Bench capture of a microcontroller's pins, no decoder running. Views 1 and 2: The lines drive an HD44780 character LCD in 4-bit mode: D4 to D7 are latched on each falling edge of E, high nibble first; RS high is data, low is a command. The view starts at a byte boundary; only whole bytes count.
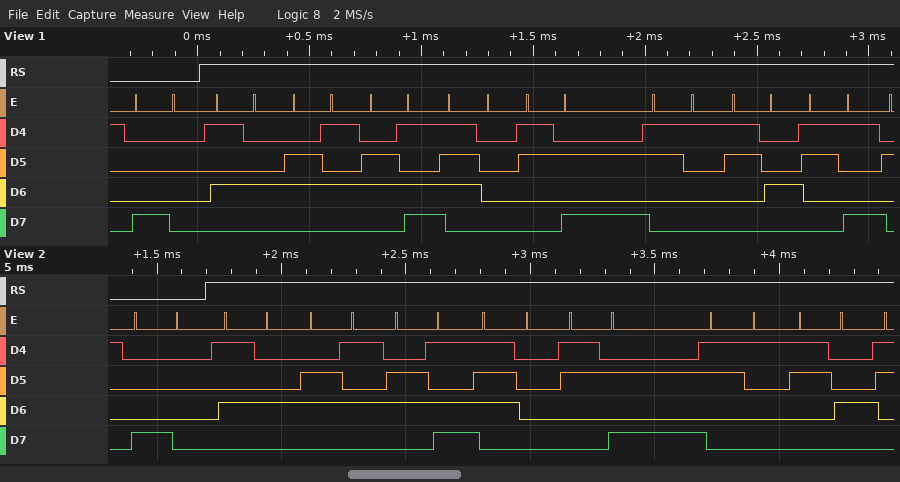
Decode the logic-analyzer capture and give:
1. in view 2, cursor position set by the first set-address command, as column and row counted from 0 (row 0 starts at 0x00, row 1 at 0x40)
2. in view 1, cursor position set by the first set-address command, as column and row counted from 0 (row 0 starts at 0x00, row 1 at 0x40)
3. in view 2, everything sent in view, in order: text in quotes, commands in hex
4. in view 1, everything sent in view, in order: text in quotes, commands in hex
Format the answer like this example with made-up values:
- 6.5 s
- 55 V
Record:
- column 0, row 0
- column 0, row 0
- 0x80 "Temp:14"
- 0x80 "Temp:149"
